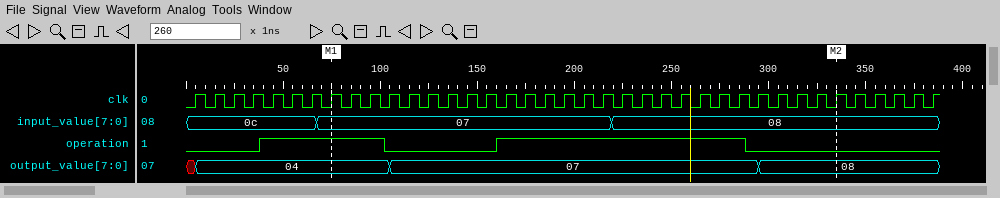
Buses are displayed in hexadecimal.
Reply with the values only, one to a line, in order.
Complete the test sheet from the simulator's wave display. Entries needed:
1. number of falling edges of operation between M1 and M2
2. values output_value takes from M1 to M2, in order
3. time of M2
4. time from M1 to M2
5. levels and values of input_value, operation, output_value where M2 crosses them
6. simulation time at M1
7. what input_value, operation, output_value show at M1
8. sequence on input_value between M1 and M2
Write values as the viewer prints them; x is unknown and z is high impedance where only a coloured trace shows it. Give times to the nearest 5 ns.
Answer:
2
04, 07, 08
335 ns
260 ns
input_value=08, operation=0, output_value=08
75 ns
input_value=07, operation=1, output_value=04
07, 08
